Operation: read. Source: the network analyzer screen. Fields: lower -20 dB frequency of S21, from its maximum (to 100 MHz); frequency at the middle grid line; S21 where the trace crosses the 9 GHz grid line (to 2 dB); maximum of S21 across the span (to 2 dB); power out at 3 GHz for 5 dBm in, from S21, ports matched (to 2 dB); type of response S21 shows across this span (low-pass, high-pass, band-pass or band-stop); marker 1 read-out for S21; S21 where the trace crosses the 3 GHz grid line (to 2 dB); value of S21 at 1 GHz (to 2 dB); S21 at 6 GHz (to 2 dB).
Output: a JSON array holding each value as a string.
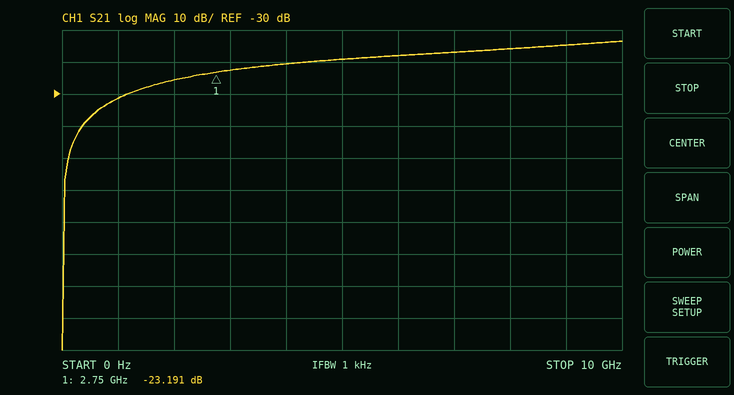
["800 MHz", "5 GHz", "-14 dB", "-14 dB", "-18 dBm", "high-pass", "-23.191 dB", "-22 dB", "-32 dB", "-18 dB"]
